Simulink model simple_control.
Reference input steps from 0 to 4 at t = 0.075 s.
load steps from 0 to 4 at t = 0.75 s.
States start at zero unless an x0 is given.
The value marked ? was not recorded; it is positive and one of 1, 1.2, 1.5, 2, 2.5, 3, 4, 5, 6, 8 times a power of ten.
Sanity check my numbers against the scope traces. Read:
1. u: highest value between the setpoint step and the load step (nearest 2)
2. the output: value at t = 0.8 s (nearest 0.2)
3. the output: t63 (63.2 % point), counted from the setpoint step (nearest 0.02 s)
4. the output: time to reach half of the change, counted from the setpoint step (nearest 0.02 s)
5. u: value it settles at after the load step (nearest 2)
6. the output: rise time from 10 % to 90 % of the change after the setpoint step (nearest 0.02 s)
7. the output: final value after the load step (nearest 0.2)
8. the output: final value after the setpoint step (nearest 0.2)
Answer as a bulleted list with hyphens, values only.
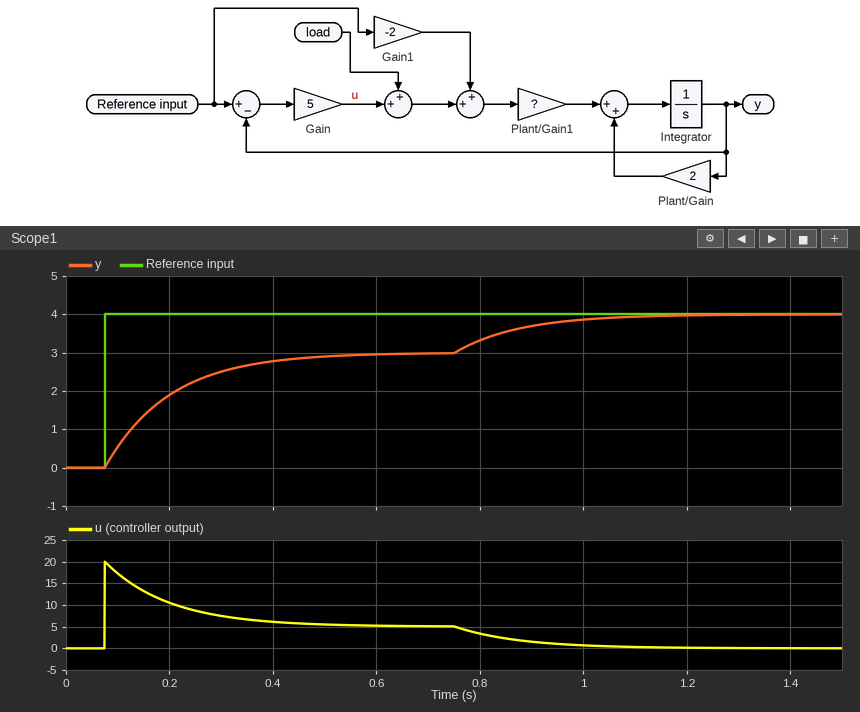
- 20
- 3.4
- 0.12 s
- 0.08 s
- 0
- 0.28 s
- 4.0
- 3.0
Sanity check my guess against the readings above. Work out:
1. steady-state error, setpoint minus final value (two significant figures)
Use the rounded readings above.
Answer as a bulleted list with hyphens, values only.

- 1.0
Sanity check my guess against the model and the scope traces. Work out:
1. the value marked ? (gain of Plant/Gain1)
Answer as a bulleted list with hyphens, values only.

- 2
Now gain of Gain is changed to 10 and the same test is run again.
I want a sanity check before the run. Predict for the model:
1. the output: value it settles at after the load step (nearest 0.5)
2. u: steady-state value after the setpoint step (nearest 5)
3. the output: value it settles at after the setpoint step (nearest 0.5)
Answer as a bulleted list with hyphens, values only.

- 4.0
- 5
- 3.5
